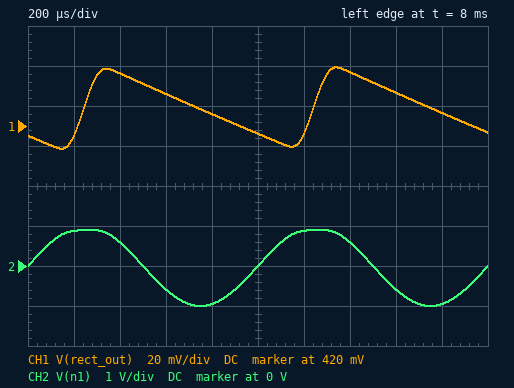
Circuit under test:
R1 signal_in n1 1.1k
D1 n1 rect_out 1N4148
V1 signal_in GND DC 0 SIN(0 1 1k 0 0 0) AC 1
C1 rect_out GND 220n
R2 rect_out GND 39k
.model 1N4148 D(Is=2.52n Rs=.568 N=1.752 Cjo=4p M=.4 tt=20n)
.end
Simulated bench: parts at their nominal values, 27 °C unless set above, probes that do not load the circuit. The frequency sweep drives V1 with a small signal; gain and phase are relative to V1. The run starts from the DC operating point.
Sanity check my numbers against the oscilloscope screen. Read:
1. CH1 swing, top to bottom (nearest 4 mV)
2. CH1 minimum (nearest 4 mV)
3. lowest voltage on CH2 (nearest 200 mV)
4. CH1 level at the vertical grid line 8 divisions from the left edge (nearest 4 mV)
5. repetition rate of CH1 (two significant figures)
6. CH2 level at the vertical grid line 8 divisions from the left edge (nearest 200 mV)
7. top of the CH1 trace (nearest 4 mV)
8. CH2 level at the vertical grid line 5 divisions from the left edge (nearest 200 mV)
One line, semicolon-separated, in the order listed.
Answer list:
40 mV; 408 mV; -1.0 V; 436 mV; 1.0 kHz; -600 mV; 448 mV; 0 V
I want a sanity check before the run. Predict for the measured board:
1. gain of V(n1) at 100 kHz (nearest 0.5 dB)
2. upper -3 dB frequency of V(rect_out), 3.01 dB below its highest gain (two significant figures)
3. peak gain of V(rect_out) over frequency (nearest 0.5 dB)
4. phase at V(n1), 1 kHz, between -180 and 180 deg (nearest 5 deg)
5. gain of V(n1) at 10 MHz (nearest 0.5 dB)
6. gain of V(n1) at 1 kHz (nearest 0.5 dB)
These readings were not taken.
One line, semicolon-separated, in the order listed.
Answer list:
0 dB; 19 Hz; -53.5 dB; 0 deg; -0.5 dB; 0 dB
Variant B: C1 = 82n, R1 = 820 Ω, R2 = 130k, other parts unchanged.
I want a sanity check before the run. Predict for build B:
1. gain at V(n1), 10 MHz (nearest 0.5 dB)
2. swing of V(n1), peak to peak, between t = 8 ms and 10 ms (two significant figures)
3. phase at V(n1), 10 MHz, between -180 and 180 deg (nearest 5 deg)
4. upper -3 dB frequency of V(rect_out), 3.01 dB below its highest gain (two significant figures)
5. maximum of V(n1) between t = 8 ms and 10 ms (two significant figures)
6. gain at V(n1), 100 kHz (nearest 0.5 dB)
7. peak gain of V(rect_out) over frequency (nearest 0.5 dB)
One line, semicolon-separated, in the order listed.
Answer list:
0 dB; 2.0 V; -10 deg; 15 Hz; 970 mV; 0 dB; -43.0 dB
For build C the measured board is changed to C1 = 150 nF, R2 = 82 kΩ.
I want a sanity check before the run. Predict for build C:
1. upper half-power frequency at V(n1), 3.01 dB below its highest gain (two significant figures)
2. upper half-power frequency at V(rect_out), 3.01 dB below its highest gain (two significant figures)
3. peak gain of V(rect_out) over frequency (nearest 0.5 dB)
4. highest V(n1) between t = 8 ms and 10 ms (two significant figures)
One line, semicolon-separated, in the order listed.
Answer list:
36 MHz; 13 Hz; -47.0 dB; 940 mV
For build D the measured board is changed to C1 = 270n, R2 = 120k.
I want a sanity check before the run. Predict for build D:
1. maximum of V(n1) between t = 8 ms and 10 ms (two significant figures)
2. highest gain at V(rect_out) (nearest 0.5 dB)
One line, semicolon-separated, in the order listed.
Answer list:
950 mV; -43.5 dB
